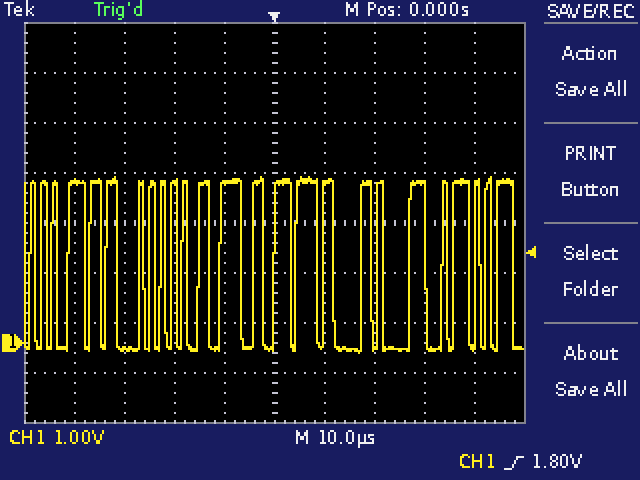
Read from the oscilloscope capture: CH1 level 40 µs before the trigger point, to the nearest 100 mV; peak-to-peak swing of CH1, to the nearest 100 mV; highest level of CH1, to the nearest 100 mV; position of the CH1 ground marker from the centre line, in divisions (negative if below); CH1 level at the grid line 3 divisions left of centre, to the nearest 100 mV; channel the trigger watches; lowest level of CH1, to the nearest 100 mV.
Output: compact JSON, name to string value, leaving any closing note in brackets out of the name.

{"CH1 level 40 µs before the trigger point, to the nearest 100 mV": "3.2 V", "peak-to-peak swing of CH1, to the nearest 100 mV": "3.5 V", "highest level of CH1, to the nearest 100 mV": "3.3 V", "position of the CH1 ground marker from the centre line, in divisions": "-2.4 div", "CH1 level at the grid line 3 divisions left of centre, to the nearest 100 mV": "-100 mV", "channel the trigger watches": "CH1", "lowest level of CH1, to the nearest 100 mV": "-200 mV"}
